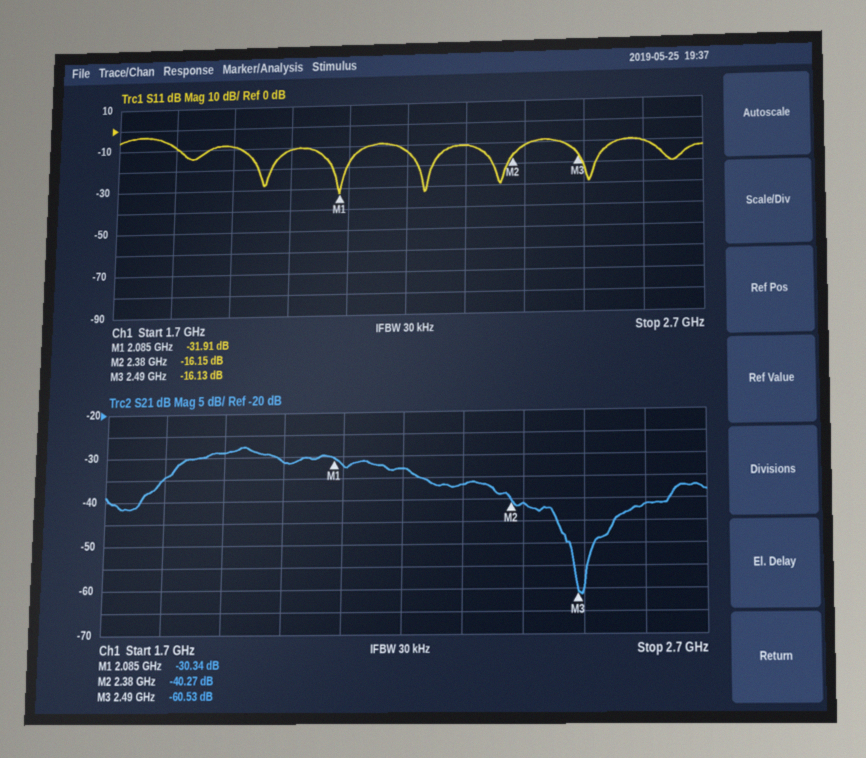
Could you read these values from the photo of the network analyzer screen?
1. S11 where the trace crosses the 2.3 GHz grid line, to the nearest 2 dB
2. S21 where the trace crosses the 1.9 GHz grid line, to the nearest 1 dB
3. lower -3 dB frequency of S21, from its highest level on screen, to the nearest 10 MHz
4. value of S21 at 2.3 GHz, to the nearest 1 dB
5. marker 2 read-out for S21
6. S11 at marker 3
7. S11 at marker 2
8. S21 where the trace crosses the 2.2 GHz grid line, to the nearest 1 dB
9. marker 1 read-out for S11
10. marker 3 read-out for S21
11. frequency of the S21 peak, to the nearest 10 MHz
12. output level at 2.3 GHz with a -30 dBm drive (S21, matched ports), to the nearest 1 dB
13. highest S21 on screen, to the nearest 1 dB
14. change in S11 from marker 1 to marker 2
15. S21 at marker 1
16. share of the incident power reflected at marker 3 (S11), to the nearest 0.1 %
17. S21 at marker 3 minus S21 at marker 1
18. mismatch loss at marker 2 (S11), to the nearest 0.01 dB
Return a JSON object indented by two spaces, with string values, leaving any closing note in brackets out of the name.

{
  "S11 where the trace crosses the 2.3 GHz grid line, to the nearest 2 dB": "-10 dB",
  "S21 where the trace crosses the 1.9 GHz grid line, to the nearest 1 dB": "-29 dB",
  "lower -3 dB frequency of S21, from its highest level on screen, to the nearest 10 MHz": "1.83 GHz",
  "value of S21 at 2.3 GHz, to the nearest 1 dB": "-37 dB",
  "marker 2 read-out for S21": "-40.27 dB",
  "S11 at marker 3": "-16.13 dB",
  "S11 at marker 2": "-16.15 dB",
  "S21 where the trace crosses the 2.2 GHz grid line, to the nearest 1 dB": "-33 dB",
  "marker 1 read-out for S11": "-31.91 dB",
  "marker 3 read-out for S21": "-60.53 dB",
  "frequency of the S21 peak, to the nearest 10 MHz": "1.93 GHz",
  "output level at 2.3 GHz with a -30 dBm drive (S21, matched ports), to the nearest 1 dB": "-67 dBm",
  "highest S21 on screen, to the nearest 1 dB": "-28 dB",
  "change in S11 from marker 1 to marker 2": "15.76 dB",
  "S21 at marker 1": "-30.34 dB",
  "share of the incident power reflected at marker 3 (S11), to the nearest 0.1 %": "2.4 %",
  "S21 at marker 3 minus S21 at marker 1": "-30.19 dB",
  "mismatch loss at marker 2 (S11), to the nearest 0.01 dB": "0.11 dB"
}
